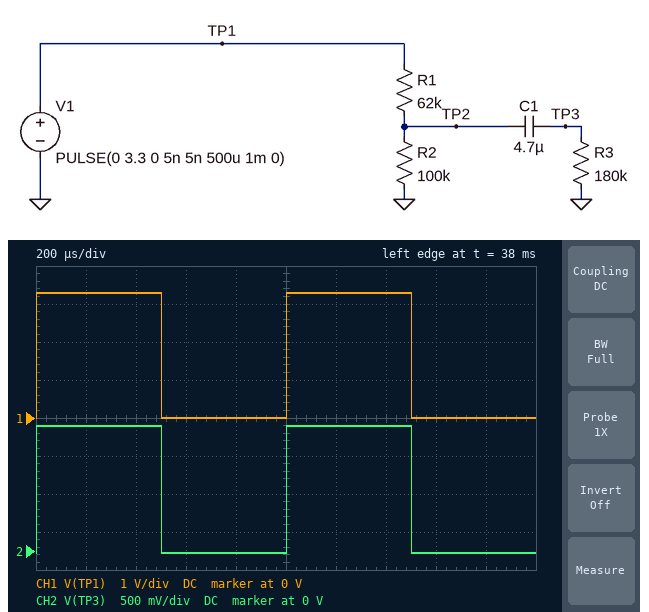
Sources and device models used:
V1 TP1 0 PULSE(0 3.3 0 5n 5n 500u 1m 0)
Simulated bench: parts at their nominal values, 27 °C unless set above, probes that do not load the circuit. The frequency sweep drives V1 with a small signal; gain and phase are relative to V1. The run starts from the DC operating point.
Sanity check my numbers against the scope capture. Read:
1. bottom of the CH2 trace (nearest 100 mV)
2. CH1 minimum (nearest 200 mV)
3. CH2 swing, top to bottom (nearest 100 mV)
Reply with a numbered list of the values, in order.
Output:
1. 0 V
2. 0 V
3. 1.7 V
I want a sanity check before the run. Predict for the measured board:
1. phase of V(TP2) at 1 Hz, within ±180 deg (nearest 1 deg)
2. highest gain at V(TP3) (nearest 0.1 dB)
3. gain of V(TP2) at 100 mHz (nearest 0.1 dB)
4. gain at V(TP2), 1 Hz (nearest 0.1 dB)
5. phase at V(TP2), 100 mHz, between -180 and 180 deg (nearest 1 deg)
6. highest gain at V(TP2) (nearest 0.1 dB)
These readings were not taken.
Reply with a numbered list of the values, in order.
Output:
1. -2 deg
2. -5.9 dB
3. -4.6 dB
4. -5.8 dB
5. -5 deg
6. -4.2 dB
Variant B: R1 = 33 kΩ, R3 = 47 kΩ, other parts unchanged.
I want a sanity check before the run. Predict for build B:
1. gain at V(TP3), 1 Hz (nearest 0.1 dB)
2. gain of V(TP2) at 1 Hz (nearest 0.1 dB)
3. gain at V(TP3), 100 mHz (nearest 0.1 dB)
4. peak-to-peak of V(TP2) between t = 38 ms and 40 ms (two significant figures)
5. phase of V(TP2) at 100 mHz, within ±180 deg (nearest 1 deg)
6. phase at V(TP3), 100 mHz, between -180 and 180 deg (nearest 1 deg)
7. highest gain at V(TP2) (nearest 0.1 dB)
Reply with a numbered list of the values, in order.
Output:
1. -7.0 dB
2. -5.2 dB
3. -19.8 dB
4. 1.6 V
5. -4 deg
6. 78 deg
7. -2.5 dB
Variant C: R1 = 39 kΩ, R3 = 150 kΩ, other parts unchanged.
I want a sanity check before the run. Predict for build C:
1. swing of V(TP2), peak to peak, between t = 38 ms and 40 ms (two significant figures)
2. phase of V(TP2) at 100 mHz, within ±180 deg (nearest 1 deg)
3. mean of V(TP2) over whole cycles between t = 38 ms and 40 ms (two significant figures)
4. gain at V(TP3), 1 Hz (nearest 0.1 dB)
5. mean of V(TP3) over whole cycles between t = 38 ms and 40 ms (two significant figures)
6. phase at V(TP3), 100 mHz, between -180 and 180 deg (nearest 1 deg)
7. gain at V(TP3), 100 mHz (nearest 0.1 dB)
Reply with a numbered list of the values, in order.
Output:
1. 2.0 V
2. -4 deg
3. 1.0 V
4. -4.5 dB
5. 950 mV
6. 62 deg
7. -11.0 dB
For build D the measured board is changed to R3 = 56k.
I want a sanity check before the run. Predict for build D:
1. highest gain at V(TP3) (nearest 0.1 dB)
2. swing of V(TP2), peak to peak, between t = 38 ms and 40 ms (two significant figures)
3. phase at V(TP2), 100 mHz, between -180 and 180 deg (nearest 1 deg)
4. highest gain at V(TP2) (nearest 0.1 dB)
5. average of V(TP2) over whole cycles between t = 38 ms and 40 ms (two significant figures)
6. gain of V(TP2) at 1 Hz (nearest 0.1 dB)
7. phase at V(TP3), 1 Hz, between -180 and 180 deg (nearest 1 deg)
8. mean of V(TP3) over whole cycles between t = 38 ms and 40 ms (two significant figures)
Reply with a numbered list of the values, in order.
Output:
1. -8.7 dB
2. 1.2 V
3. -6 deg
4. -4.2 dB
5. 640 mV
6. -7.9 dB
7. 20 deg
8. 550 mV
